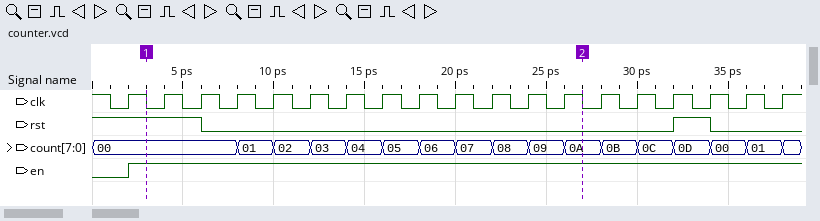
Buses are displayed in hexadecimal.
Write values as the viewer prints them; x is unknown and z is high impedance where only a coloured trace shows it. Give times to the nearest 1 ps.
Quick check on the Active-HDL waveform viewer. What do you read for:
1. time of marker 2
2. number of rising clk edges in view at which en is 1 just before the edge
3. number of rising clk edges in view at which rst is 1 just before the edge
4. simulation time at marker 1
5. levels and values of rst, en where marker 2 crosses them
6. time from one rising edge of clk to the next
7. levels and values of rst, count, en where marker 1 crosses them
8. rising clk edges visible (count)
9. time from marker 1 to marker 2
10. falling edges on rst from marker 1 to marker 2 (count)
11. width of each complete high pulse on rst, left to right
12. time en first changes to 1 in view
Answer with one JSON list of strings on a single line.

["27 ps", "18", "4", "3 ps", "rst=0, en=1", "2 ps", "rst=1, count=00, en=1", "19", "24 ps", "1", "2 ps", "2 ps"]
